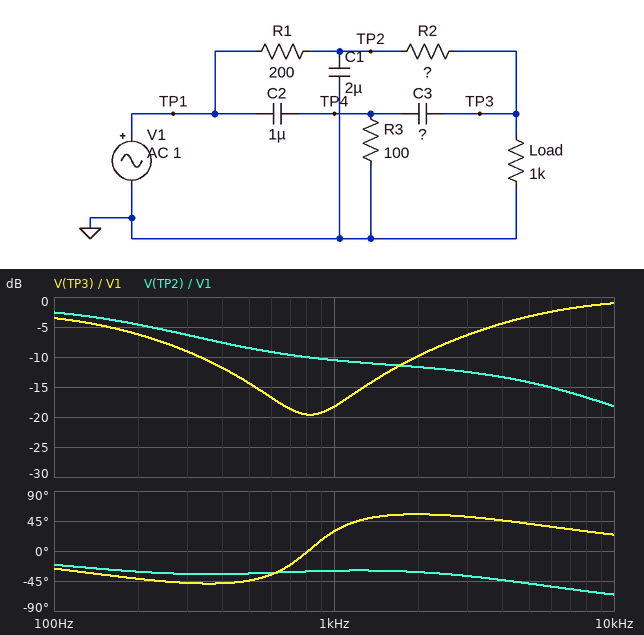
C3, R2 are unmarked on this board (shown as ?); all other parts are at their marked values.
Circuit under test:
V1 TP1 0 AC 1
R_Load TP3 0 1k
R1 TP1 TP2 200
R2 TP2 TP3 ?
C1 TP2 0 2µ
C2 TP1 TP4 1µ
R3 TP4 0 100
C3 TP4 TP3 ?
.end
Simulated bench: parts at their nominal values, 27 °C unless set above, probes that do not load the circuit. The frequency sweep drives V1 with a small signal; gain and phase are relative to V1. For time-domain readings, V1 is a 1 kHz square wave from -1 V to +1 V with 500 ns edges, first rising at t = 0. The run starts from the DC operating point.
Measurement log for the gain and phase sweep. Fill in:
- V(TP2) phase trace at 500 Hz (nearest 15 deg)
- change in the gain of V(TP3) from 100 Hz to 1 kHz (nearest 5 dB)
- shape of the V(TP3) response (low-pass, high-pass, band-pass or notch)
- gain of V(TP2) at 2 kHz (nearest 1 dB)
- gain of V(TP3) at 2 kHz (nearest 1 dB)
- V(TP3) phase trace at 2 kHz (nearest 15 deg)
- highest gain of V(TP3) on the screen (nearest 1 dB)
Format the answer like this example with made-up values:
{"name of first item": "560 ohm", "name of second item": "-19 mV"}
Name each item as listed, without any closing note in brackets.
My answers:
{"V(TP2) phase trace at 500 Hz": "-30 deg", "change in the gain of V(TP3) from 100 Hz to 1 kHz": "-15 dB", "shape of the V(TP3) response": "notch", "gain of V(TP2) at 2 kHz": "-12 dB", "gain of V(TP3) at 2 kHz": "-10 dB", "V(TP3) phase trace at 2 kHz": "60 deg", "highest gain of V(TP3) on the screen": "-1 dB"}
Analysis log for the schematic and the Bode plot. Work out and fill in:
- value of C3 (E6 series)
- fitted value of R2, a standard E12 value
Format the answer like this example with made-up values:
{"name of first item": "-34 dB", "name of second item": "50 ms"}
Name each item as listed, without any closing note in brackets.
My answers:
{"value of C3": "2.2 µF", "fitted value of R2, a standard E12 value": "82 Ω"}
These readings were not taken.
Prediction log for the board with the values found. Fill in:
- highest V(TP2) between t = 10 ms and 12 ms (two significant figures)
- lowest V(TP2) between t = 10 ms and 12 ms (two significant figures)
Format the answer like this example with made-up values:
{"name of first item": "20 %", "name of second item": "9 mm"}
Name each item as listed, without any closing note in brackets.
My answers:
{"highest V(TP2) between t = 10 ms and 12 ms": "410 mV", "lowest V(TP2) between t = 10 ms and 12 ms": "-410 mV"}
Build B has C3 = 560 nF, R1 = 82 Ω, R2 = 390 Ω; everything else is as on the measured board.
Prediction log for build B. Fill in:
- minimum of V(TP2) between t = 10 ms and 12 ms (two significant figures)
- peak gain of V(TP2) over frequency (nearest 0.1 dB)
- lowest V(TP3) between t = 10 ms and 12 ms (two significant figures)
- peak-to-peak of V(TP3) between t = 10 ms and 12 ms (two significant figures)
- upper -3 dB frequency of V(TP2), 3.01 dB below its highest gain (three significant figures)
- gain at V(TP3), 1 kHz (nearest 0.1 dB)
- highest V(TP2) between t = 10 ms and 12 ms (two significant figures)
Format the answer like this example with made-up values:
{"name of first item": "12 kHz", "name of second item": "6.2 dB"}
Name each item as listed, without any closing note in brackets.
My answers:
{"minimum of V(TP2) between t = 10 ms and 12 ms": "-820 mV", "peak gain of V(TP2) over frequency": "-0.5 dB", "lowest V(TP3) between t = 10 ms and 12 ms": "-1.6 V", "peak-to-peak of V(TP3) between t = 10 ms and 12 ms": "3.3 V", "upper -3 dB frequency of V(TP2), 3.01 dB below its highest gain": "878 Hz", "gain at V(TP3), 1 kHz": "-32.7 dB", "highest V(TP2) between t = 10 ms and 12 ms": "820 mV"}
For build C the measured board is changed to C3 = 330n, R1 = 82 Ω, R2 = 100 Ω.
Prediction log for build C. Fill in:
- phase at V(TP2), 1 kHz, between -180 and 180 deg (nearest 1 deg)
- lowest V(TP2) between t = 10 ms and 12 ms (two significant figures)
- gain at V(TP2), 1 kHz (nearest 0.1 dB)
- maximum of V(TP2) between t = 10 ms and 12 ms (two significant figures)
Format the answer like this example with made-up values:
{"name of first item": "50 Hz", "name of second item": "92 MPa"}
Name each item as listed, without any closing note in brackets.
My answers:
{"phase at V(TP2), 1 kHz, between -180 and 180 deg": "-43 deg", "lowest V(TP2) between t = 10 ms and 12 ms": "-810 mV", "gain at V(TP2), 1 kHz": "-4.5 dB", "maximum of V(TP2) between t = 10 ms and 12 ms": "810 mV"}
